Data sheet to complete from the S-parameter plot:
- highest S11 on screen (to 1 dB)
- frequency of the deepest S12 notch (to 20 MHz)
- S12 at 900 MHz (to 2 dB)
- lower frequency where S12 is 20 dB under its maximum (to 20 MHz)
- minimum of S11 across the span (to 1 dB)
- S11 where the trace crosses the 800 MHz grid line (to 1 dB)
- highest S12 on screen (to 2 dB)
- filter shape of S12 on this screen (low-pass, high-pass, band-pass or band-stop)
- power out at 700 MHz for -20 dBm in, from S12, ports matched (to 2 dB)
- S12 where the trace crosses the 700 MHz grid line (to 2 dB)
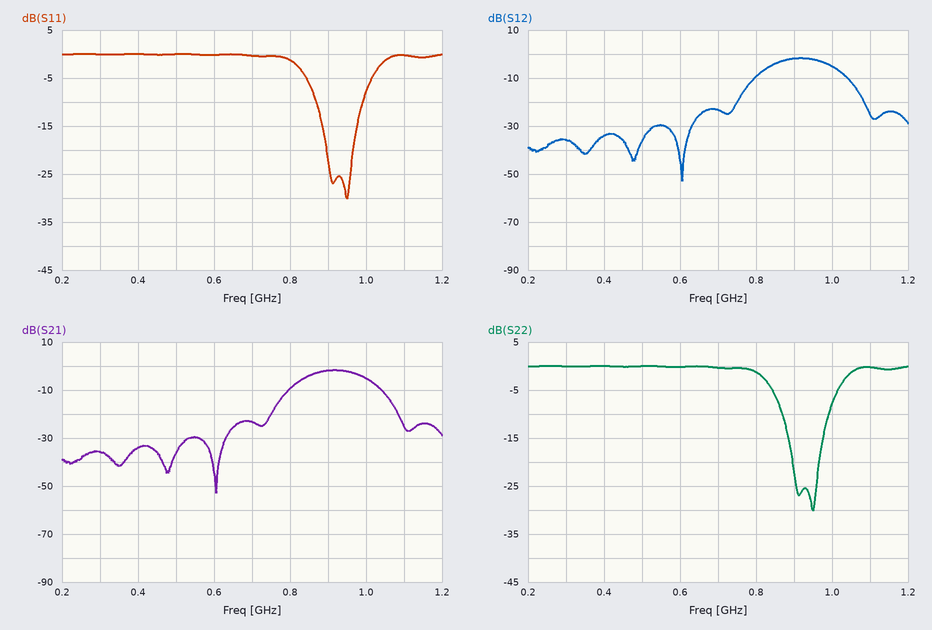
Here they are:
0 dB
600 MHz
-2 dB
740 MHz
-30 dB
-1 dB
-2 dB
band-pass
-44 dBm
-24 dB
